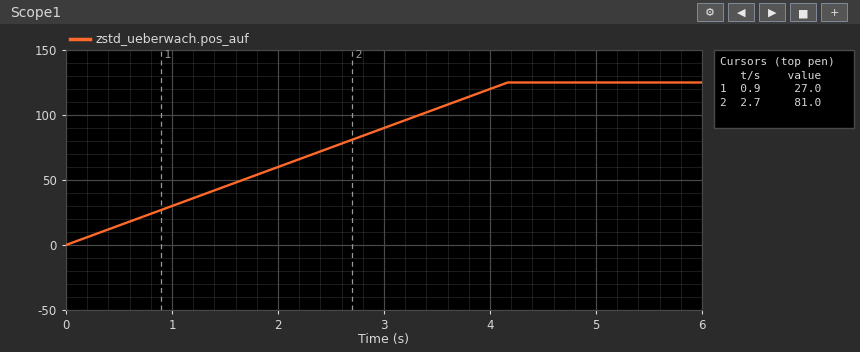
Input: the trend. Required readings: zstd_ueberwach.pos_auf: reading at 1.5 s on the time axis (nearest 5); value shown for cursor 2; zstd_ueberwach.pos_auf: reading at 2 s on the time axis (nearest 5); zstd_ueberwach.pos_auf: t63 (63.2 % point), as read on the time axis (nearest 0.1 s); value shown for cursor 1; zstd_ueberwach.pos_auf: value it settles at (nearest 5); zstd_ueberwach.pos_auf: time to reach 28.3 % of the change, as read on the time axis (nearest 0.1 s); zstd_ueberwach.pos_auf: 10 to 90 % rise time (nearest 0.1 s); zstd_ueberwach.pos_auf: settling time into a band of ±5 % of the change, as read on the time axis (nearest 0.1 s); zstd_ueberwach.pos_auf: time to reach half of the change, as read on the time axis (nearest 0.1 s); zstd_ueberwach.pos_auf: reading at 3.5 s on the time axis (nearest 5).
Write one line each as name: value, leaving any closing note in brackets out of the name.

zstd_ueberwach.pos_auf: reading at 1.5 s on the time axis: 45
value shown for cursor 2: 81.0
zstd_ueberwach.pos_auf: reading at 2 s on the time axis: 60
zstd_ueberwach.pos_auf: t63 (63.2 % point), as read on the time axis: 2.6 s
value shown for cursor 1: 27.0
zstd_ueberwach.pos_auf: value it settles at: 125
zstd_ueberwach.pos_auf: time to reach 28.3 % of the change, as read on the time axis: 1.2 s
zstd_ueberwach.pos_auf: 10 to 90 % rise time: 3.3 s
zstd_ueberwach.pos_auf: settling time into a band of ±5 % of the change, as read on the time axis: 4.0 s
zstd_ueberwach.pos_auf: time to reach half of the change, as read on the time axis: 2.1 s
zstd_ueberwach.pos_auf: reading at 3.5 s on the time axis: 105
